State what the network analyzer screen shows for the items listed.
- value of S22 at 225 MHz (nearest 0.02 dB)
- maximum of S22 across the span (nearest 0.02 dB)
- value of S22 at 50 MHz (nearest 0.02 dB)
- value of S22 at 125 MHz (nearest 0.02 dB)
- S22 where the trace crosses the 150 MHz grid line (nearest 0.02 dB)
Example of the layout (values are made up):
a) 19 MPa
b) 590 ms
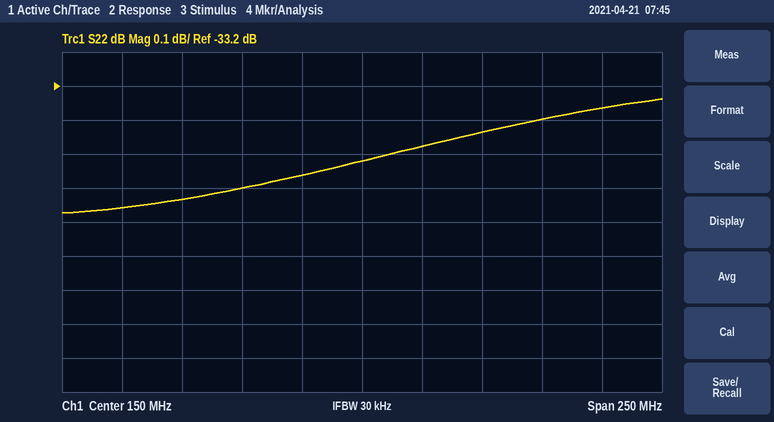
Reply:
a) -33.30 dB
b) -33.24 dB
c) -33.56 dB
d) -33.46 dB
e) -33.42 dB
